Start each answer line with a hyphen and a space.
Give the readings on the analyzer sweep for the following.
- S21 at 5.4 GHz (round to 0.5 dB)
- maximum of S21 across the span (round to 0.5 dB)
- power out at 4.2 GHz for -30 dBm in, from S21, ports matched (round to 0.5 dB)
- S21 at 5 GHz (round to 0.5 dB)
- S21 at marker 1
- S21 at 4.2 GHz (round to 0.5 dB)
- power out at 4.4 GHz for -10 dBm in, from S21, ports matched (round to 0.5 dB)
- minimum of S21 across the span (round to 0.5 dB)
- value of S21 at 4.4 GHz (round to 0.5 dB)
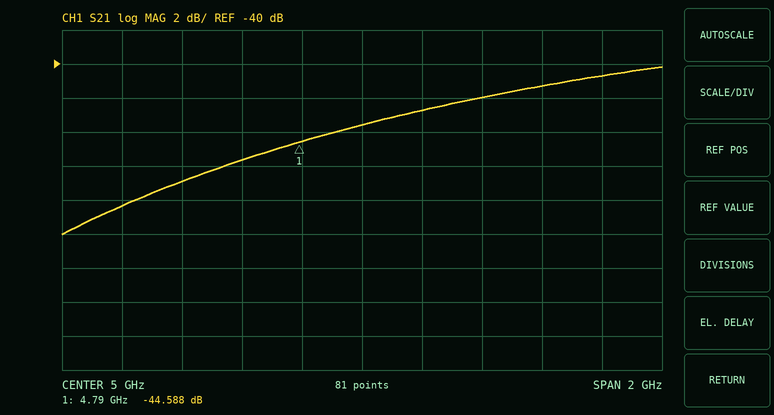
- -42.0 dB
- -40.0 dB
- -78.5 dBm
- -43.5 dB
- -44.588 dB
- -48.5 dB
- -57.0 dBm
- -50.0 dB
- -47.0 dB
